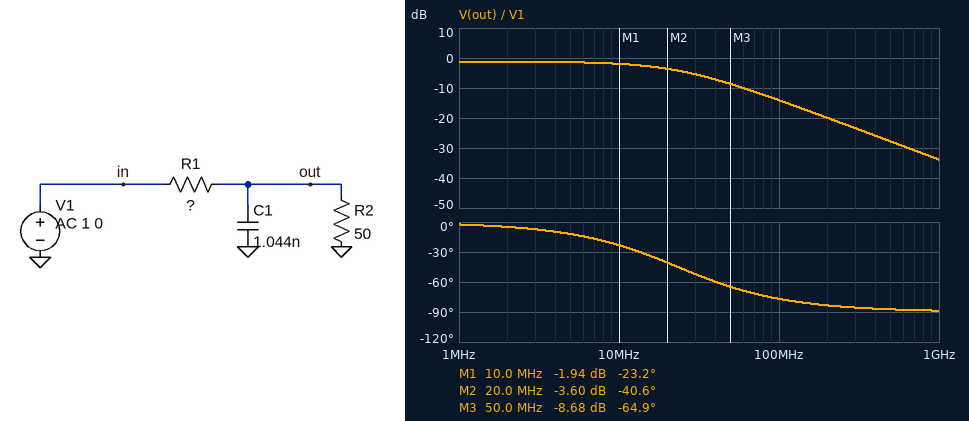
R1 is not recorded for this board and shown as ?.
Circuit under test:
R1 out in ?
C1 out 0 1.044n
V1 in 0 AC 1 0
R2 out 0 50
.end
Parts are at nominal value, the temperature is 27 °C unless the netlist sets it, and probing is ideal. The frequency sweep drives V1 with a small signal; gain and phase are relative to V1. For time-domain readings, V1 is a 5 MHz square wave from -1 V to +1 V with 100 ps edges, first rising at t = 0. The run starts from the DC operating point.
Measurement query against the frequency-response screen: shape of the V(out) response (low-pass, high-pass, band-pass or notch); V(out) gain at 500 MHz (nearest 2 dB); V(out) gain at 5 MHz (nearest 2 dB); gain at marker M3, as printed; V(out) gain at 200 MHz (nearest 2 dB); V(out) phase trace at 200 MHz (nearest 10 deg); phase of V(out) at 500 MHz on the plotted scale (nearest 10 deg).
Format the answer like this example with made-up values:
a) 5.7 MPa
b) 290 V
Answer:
a) low-pass
b) -28 dB
c) -2 dB
d) -8.68 dB
e) -20 dB
f) -80 deg
g) -90 deg
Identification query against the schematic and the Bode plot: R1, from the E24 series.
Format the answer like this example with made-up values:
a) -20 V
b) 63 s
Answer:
a) 7.5 Ω
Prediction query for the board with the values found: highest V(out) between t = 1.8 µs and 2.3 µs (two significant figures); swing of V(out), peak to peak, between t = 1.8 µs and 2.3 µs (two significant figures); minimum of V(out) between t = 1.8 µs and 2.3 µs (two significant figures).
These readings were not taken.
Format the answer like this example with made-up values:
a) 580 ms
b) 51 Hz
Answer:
a) 870 mV
b) 1.7 V
c) -870 mV
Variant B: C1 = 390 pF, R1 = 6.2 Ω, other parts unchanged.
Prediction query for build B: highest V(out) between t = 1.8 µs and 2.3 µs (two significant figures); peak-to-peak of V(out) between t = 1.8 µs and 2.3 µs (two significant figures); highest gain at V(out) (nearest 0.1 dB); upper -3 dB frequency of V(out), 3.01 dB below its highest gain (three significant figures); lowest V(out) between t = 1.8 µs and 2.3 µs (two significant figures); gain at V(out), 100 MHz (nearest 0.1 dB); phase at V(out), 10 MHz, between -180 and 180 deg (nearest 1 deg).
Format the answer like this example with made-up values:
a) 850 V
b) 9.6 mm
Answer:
a) 890 mV
b) 1.8 V
c) -1.0 dB
d) 74.0 MHz
e) -890 mV
f) -5.5 dB
g) -8 deg
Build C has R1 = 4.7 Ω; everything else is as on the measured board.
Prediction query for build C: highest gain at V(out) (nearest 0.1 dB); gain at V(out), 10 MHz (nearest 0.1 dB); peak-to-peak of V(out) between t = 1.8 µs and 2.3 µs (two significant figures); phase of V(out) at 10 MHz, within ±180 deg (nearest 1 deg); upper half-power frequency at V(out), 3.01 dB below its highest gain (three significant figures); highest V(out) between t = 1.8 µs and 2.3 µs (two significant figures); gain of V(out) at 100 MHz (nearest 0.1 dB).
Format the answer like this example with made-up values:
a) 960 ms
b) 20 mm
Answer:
a) -0.8 dB
b) -1.1 dB
c) 1.8 V
d) -16 deg
e) 35.5 MHz
f) 910 mV
g) -10.3 dB
